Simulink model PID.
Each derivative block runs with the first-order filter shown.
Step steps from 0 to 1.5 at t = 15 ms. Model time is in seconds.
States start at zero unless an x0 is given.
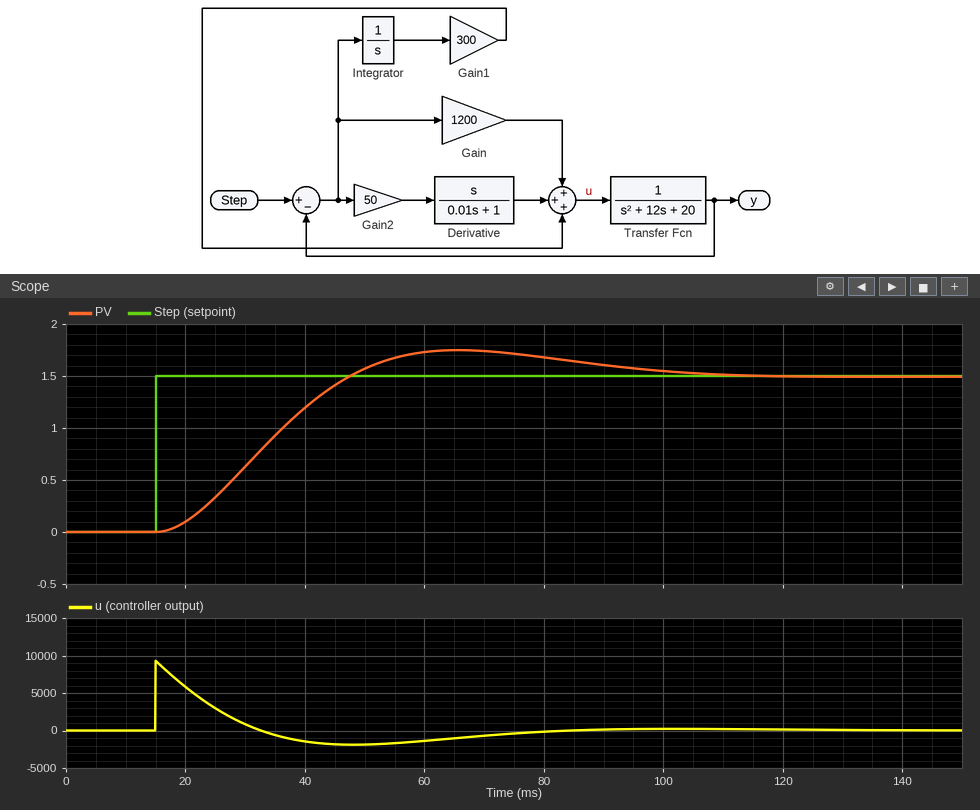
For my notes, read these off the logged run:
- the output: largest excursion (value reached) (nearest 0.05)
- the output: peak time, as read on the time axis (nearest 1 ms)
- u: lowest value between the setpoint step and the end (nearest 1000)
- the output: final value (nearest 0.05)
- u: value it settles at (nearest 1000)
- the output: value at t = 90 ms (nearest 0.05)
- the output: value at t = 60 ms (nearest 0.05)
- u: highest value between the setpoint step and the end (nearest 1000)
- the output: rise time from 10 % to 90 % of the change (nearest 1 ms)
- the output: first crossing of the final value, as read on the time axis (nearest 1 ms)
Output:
1.75
66 ms
-2000
1.50
0
1.60
1.75
9000
22 ms
47 ms
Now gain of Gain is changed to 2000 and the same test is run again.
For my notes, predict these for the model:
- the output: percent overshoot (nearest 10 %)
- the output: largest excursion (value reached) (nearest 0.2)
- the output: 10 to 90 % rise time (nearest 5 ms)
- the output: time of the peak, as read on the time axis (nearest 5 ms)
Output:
30 %
2.0
20 ms
60 ms
